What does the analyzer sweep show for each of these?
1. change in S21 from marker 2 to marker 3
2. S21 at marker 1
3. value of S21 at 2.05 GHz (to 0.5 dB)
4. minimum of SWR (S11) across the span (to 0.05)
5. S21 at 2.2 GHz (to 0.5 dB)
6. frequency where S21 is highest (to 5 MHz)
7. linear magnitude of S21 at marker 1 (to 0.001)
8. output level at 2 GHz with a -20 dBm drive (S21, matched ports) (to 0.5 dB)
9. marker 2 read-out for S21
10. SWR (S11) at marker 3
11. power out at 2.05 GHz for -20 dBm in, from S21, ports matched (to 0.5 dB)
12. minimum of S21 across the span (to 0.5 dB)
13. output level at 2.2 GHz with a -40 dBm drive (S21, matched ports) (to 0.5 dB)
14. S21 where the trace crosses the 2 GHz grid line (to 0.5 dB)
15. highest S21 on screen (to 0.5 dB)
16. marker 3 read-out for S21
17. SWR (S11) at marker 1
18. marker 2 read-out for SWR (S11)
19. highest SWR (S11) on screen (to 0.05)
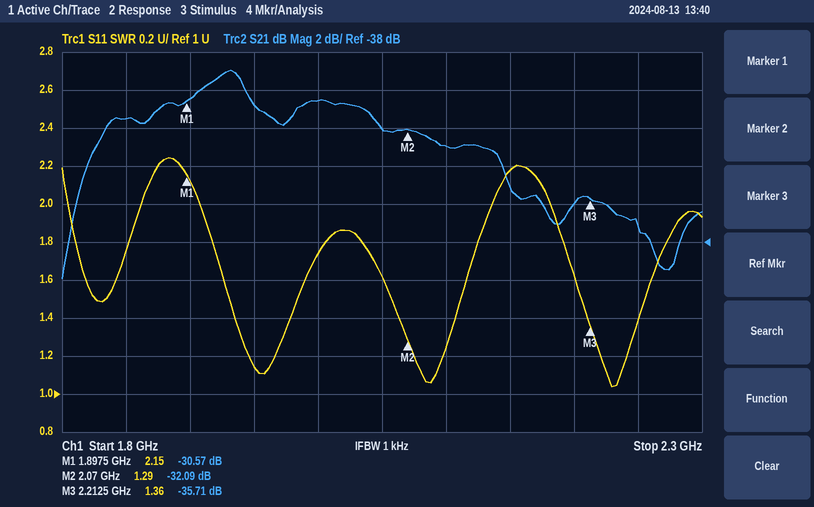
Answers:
-3.62 dB
-30.57 dB
-32.0 dB
1.05
-36.0 dB
1.930 GHz
0.030
-50.5 dBm
-32.09 dB
1.36
-52.0 dBm
-40.0 dB
-76.0 dBm
-30.5 dB
-29.0 dB
-35.71 dB
2.15
1.29
2.25
